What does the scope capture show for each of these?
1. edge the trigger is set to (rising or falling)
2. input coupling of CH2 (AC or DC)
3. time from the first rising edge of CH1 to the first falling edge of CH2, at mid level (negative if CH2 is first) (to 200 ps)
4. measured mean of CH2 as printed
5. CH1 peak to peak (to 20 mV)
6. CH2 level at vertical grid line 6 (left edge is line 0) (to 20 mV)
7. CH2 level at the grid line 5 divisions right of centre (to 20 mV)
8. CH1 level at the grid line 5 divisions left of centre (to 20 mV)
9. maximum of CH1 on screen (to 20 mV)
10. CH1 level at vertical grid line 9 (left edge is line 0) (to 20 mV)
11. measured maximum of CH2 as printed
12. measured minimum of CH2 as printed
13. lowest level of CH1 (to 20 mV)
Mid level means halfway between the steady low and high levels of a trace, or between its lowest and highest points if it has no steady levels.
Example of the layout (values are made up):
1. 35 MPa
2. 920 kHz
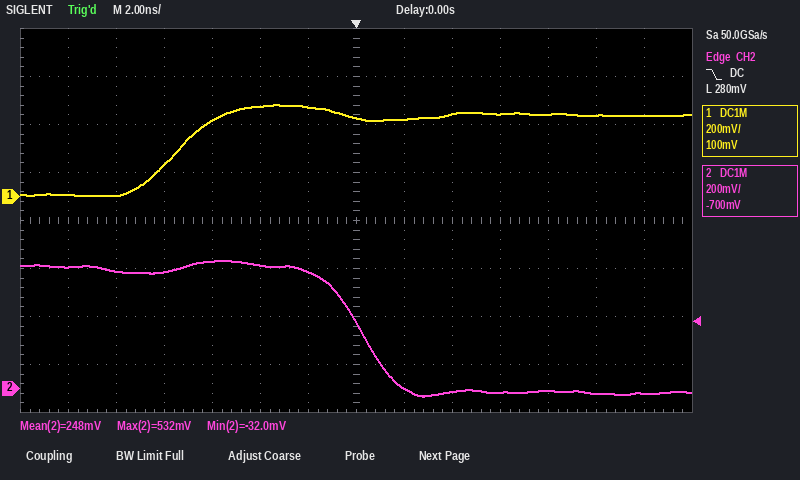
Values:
1. falling
2. DC
3. +7.6 ns
4. 248 mV
5. 380 mV
6. 480 mV
7. -20 mV
8. 0 mV
9. 380 mV
10. 340 mV
11. 532 mV
12. -32.0 mV
13. 0 mV
